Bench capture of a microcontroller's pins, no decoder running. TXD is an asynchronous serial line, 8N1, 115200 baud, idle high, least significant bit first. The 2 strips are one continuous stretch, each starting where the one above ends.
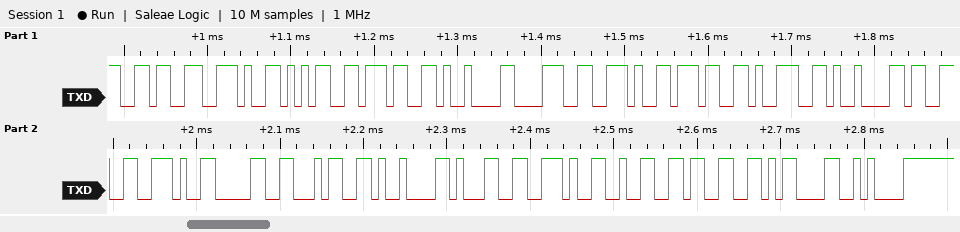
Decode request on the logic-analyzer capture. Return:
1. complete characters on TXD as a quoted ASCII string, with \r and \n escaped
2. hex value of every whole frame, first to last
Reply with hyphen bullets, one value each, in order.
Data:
- "6.57\t8.79\t3.04\t1.23\r\n"
- 0x36 0x2E 0x35 0x37 0x09 0x38 0x2E 0x37 0x39 0x09 0x33 0x2E 0x30 0x34 0x09 0x31 0x2E 0x32 0x33 0x0D 0x0A
